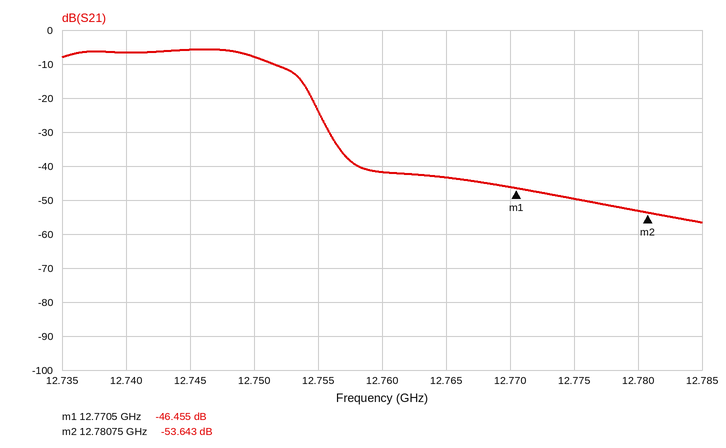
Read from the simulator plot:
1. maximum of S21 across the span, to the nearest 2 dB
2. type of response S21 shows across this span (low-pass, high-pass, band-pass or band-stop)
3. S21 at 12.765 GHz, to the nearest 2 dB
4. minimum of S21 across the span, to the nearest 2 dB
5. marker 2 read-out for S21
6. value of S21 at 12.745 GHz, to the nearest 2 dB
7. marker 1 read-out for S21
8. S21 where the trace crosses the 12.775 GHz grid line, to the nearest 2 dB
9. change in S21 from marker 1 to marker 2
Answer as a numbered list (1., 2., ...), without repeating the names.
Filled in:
1. -6 dB
2. low-pass
3. -44 dB
4. -56 dB
5. -53.643 dB
6. -6 dB
7. -46.455 dB
8. -50 dB
9. -7.188 dB
